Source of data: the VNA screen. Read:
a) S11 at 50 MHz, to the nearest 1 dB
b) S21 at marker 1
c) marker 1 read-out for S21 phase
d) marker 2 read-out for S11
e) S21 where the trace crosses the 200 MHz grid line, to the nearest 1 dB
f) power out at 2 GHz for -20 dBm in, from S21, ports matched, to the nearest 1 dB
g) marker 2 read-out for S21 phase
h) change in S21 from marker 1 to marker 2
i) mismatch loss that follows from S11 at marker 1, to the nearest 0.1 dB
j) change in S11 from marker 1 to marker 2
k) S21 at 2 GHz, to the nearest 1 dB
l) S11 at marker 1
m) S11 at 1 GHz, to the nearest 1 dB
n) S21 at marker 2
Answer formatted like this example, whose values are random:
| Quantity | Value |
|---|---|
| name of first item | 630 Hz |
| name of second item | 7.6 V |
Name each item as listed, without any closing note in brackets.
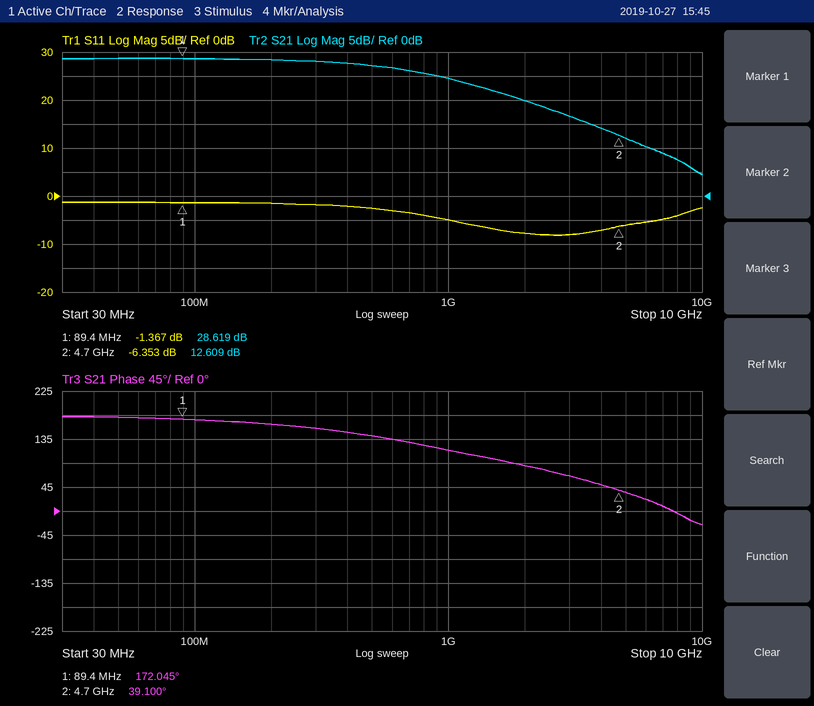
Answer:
| Quantity | Value |
|---|---|
| S11 at 50 MHz, to the nearest 1 dB | -1 dB |
| S21 at marker 1 | 28.619 dB |
| marker 1 read-out for S21 phase | 172.045° |
| marker 2 read-out for S11 | -6.353 dB |
| S21 where the trace crosses the 200 MHz grid line, to the nearest 1 dB | 28 dB |
| power out at 2 GHz for -20 dBm in, from S21, ports matched, to the nearest 1 dB | 0 dBm |
| marker 2 read-out for S21 phase | 39.100° |
| change in S21 from marker 1 to marker 2 | -16.010 dB |
| mismatch loss that follows from S11 at marker 1, to the nearest 0.1 dB | 5.7 dB |
| change in S11 from marker 1 to marker 2 | -4.986 dB |
| S21 at 2 GHz, to the nearest 1 dB | 20 dB |
| S11 at marker 1 | -1.367 dB |
| S11 at 1 GHz, to the nearest 1 dB | -5 dB |
| S21 at marker 2 | 12.609 dB |
